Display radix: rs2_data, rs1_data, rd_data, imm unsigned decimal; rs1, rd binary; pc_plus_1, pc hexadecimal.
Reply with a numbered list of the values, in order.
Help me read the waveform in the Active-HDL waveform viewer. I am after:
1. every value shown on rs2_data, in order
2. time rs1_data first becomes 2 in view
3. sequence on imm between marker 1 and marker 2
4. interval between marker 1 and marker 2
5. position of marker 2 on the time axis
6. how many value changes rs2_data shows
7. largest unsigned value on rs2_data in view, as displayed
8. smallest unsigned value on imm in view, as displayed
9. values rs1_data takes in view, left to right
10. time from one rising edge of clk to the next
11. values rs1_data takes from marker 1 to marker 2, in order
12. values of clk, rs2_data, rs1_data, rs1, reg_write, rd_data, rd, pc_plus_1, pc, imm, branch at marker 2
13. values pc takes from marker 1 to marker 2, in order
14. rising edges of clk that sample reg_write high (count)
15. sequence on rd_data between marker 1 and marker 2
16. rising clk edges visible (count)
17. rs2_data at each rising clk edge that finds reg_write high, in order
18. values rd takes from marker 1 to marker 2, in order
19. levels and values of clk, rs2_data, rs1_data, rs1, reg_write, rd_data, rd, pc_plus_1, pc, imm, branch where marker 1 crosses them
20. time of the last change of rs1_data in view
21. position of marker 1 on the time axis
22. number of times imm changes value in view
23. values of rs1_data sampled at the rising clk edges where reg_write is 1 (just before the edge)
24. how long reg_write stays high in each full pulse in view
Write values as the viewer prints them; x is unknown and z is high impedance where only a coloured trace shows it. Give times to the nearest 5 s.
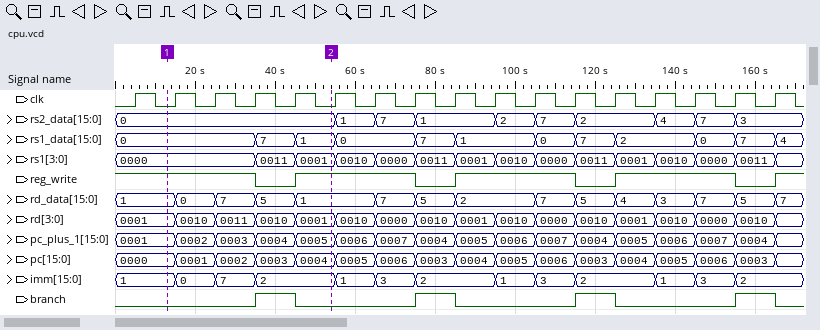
1. 0, 1, 7, 1, 2, 7, 2, 4, 7, 3
2. 125 s
3. 1, 0, 7, 2
4. 40 s
5. 55 s
6. 9
7. 7
8. 0
9. 0, 7, 1, 0, 7, 1, 0, 7, 2, 0, 7, 4
10. 10 s
11. 0, 7, 1
12. clk=0, rs2_data=0, rs1_data=1, rs1=0001, reg_write=1, rd_data=1, rd=0001, pc_plus_1=0005, pc=0004, imm=2, branch=0
13. 0000, 0001, 0002, 0003, 0004
14. 13
15. 1, 0, 7, 5, 1
16. 17
17. 0, 0, 0, 0, 0, 1, 7, 1, 2, 7, 2, 4, 7
18. 0001, 0010, 0011, 0010, 0001
19. clk=0, rs2_data=0, rs1_data=0, rs1=0000, reg_write=1, rd_data=1, rd=0001, pc_plus_1=0001, pc=0000, imm=1, branch=0
20. 165 s
21. 15 s
22. 12
23. 0, 0, 0, 0, 1, 0, 0, 1, 1, 0, 2, 2, 0
24. 30 s, 30 s, 30 s
